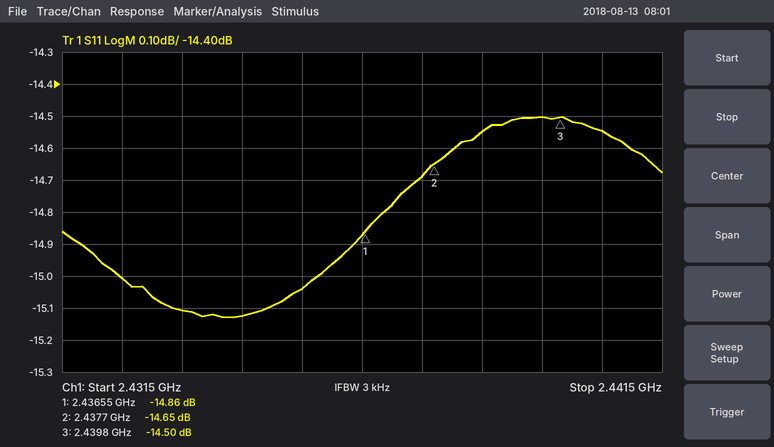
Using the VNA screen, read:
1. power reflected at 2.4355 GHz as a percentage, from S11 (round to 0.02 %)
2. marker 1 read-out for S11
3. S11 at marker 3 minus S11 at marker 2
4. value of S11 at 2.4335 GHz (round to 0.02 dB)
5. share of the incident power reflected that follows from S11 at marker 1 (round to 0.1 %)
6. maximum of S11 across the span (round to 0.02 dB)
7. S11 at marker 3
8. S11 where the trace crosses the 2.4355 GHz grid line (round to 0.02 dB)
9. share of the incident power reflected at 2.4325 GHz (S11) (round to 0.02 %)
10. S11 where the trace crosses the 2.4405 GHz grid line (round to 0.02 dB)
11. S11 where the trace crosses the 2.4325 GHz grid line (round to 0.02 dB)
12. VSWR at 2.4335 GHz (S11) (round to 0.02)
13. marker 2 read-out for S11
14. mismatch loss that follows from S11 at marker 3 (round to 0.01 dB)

3.14 %
-14.86 dB
0.15 dB
-15.10 dB
3.3 %
-14.50 dB
-14.50 dB
-15.04 dB
3.16 %
-14.54 dB
-15.00 dB
1.42
-14.65 dB
0.16 dB
